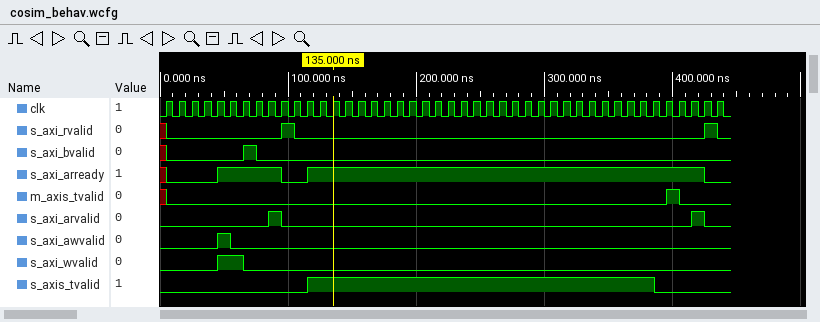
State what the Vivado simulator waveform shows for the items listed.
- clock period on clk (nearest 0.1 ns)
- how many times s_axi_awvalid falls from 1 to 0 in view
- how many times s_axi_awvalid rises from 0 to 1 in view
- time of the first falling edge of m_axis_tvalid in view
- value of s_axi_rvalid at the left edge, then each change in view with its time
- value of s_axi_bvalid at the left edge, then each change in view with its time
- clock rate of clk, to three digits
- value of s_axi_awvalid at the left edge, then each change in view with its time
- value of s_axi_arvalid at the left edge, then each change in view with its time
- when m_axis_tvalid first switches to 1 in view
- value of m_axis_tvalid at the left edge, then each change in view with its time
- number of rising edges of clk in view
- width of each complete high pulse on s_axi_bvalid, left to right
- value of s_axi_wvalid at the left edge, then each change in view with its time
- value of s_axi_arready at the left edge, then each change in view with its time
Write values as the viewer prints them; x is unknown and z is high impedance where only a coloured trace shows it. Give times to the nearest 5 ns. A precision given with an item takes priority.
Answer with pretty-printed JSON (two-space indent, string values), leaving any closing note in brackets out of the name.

{
  "clock period on clk": "10 ns",
  "how many times s_axi_awvalid falls from 1 to 0 in view": "1",
  "how many times s_axi_awvalid rises from 0 to 1 in view": "1",
  "time of the first falling edge of m_axis_tvalid in view": "405 ns",
  "value of s_axi_rvalid at the left edge, then each change in view with its time": "x, 0 at 5 ns, 1 at 95 ns, 0 at 105 ns, 1 at 425 ns, 0 at 435 ns",
  "value of s_axi_bvalid at the left edge, then each change in view with its time": "x, 0 at 5 ns, 1 at 65 ns, 0 at 75 ns",
  "clock rate of clk, to three digits": "100 MHz",
  "value of s_axi_awvalid at the left edge, then each change in view with its time": "0, 1 at 45 ns, 0 at 55 ns",
  "value of s_axi_arvalid at the left edge, then each change in view with its time": "0, 1 at 85 ns, 0 at 95 ns, 1 at 415 ns, 0 at 425 ns",
  "when m_axis_tvalid first switches to 1 in view": "395 ns",
  "value of m_axis_tvalid at the left edge, then each change in view with its time": "x, 0 at 5 ns, 1 at 395 ns, 0 at 405 ns",
  "number of rising edges of clk in view": "44",
  "width of each complete high pulse on s_axi_bvalid, left to right": "10 ns",
  "value of s_axi_wvalid at the left edge, then each change in view with its time": "0, 1 at 45 ns, 0 at 65 ns",
  "value of s_axi_arready at the left edge, then each change in view with its time": "x, 0 at 5 ns, 1 at 45 ns, 0 at 95 ns, 1 at 115 ns, 0 at 425 ns"
}
